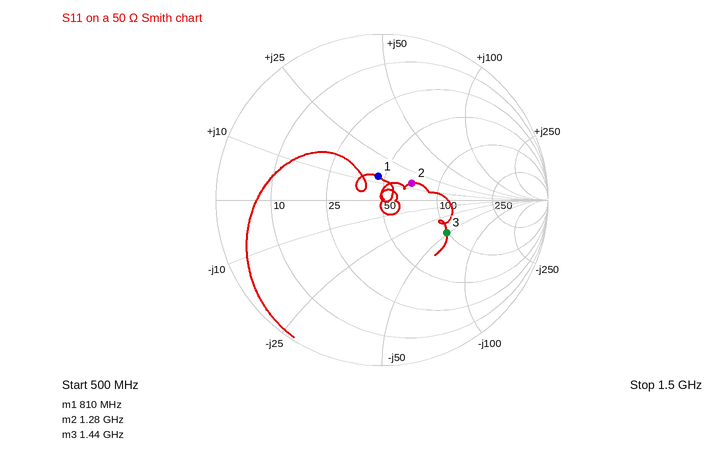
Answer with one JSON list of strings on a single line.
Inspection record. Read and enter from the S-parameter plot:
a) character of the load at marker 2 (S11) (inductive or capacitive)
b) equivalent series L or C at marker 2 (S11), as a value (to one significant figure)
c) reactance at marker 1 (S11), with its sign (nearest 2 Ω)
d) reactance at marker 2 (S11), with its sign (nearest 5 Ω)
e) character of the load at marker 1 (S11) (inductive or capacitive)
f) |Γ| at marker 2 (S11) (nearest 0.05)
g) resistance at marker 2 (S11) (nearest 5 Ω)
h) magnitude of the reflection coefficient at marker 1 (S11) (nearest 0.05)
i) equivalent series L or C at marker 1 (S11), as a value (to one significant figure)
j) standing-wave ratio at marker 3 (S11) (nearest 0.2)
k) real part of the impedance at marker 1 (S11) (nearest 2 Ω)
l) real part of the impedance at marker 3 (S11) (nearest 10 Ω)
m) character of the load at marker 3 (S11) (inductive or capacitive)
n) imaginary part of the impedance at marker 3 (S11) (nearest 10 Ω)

["inductive", "2 nH", "+14 Ω", "+15 Ω", "inductive", "0.20", "70 Ω", "0.15", "3 nH", "2.6", "46 Ω", "100 Ω", "capacitive", "-50 Ω"]
